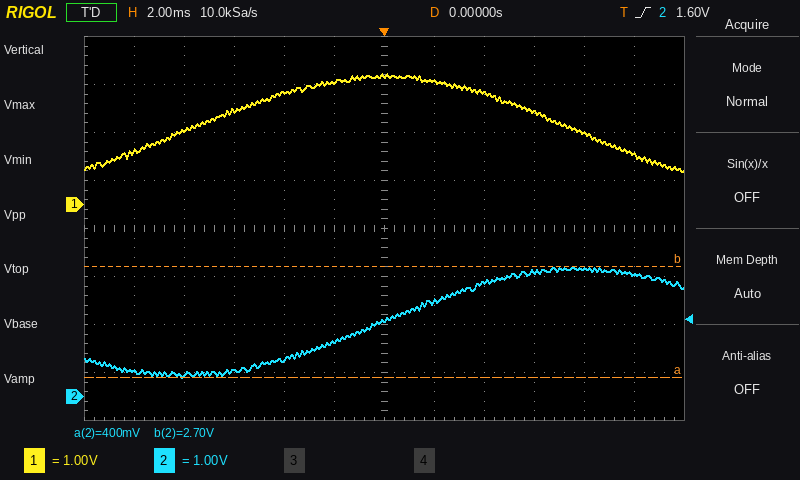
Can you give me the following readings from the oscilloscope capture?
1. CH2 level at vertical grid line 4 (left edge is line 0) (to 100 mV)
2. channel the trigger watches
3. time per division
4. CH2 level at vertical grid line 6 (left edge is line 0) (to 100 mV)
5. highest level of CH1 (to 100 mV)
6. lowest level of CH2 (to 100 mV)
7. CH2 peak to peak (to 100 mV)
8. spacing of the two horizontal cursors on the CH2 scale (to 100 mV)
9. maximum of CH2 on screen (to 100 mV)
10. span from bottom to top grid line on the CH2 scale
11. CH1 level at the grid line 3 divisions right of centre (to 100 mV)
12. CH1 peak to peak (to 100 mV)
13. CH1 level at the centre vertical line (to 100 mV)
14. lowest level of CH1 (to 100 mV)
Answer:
800 mV
CH2
2 ms
1.6 V
2.7 V
400 mV
2.3 V
2.3 V
2.7 V
8 V
1.9 V
2.0 V
2.7 V
700 mV
